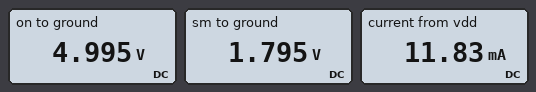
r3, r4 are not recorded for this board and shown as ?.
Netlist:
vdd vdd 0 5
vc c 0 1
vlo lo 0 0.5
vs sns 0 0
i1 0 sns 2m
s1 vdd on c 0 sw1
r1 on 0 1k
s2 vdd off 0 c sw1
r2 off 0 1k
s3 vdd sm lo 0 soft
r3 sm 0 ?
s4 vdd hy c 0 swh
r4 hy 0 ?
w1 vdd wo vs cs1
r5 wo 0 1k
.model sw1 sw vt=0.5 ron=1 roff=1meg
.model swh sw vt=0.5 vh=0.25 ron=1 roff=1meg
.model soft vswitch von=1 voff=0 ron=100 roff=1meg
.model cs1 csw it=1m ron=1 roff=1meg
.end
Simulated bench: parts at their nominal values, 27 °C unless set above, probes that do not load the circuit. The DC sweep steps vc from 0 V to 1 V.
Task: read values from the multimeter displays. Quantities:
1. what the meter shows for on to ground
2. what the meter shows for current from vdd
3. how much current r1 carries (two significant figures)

4.995 V
11.83 mA
5.0 mA
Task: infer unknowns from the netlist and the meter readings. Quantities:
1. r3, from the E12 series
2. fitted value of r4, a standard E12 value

5.6 kΩ
3.3 kΩ
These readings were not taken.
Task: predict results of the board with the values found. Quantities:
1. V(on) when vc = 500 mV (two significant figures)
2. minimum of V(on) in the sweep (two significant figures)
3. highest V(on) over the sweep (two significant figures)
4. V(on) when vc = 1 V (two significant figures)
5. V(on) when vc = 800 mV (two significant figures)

5.0 V
5.0 mV
5.0 V
5.0 V
5.0 V
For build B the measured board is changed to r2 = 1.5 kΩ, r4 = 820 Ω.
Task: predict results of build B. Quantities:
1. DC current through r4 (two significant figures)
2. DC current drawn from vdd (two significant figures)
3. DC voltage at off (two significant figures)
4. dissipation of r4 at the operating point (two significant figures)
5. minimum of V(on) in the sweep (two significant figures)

6.1 mA
16 mA
7.5 mV
30 mW
5.0 mV
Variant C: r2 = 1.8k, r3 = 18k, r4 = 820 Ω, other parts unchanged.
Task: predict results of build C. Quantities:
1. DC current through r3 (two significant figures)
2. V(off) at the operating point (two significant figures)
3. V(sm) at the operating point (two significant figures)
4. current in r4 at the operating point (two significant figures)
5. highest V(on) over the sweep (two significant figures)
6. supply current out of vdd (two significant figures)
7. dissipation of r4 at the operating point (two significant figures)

180 µA
9.0 mV
3.2 V
6.1 mA
5.0 V
16 mA
30 mW
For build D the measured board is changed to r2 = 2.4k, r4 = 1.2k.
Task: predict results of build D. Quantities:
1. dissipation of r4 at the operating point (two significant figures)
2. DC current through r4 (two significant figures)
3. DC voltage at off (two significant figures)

21 mW
4.2 mA
12 mV
